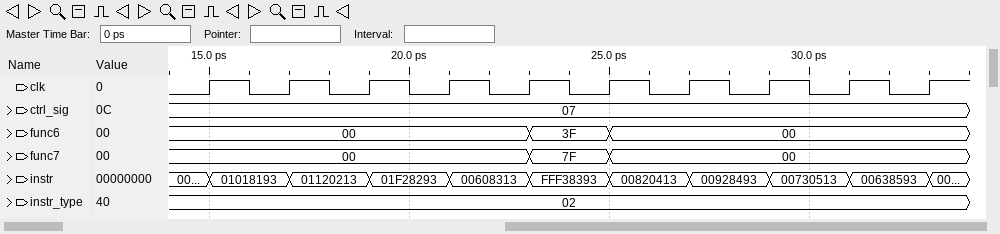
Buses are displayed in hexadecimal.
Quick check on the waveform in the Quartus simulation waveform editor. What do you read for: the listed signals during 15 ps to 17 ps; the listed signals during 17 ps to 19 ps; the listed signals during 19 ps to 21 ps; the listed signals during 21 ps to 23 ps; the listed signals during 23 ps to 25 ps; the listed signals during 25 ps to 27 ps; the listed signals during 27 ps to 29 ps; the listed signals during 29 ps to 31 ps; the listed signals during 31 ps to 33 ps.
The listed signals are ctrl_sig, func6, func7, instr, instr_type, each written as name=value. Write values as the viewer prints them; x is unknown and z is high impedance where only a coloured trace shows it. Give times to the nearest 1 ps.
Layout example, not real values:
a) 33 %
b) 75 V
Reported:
a) ctrl_sig=07, func6=00, func7=00, instr=01018193, instr_type=02
b) ctrl_sig=07, func6=00, func7=00, instr=01120213, instr_type=02
c) ctrl_sig=07, func6=00, func7=00, instr=01F28293, instr_type=02
d) ctrl_sig=07, func6=00, func7=00, instr=00608313, instr_type=02
e) ctrl_sig=07, func6=3F, func7=7F, instr=FFF38393, instr_type=02
f) ctrl_sig=07, func6=00, func7=00, instr=00820413, instr_type=02
g) ctrl_sig=07, func6=00, func7=00, instr=00928493, instr_type=02
h) ctrl_sig=07, func6=00, func7=00, instr=00730513, instr_type=02
i) ctrl_sig=07, func6=00, func7=00, instr=00638593, instr_type=02
